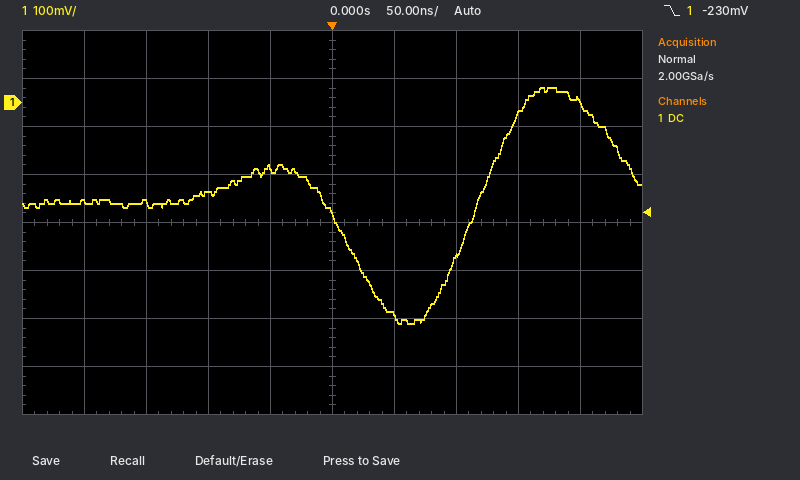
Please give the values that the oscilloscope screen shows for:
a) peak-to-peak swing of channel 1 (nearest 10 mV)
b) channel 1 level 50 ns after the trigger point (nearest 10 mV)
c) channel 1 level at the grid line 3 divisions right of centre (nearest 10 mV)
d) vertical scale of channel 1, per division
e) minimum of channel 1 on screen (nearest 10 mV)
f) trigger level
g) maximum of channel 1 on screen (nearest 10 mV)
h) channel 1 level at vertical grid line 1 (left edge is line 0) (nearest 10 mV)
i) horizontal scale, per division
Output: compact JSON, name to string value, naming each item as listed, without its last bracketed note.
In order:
{"peak-to-peak swing of channel 1": "490 mV", "channel 1 level 50 ns after the trigger point": "-440 mV", "channel 1 level at the grid line 3 divisions right of centre": "-30 mV", "vertical scale of channel 1, per division": "100 mV", "minimum of channel 1 on screen": "-460 mV", "trigger level": "-230 mV", "maximum of channel 1 on screen": "30 mV", "channel 1 level at vertical grid line 1 (left edge is line 0)": "-210 mV", "horizontal scale, per division": "50 ns"}
